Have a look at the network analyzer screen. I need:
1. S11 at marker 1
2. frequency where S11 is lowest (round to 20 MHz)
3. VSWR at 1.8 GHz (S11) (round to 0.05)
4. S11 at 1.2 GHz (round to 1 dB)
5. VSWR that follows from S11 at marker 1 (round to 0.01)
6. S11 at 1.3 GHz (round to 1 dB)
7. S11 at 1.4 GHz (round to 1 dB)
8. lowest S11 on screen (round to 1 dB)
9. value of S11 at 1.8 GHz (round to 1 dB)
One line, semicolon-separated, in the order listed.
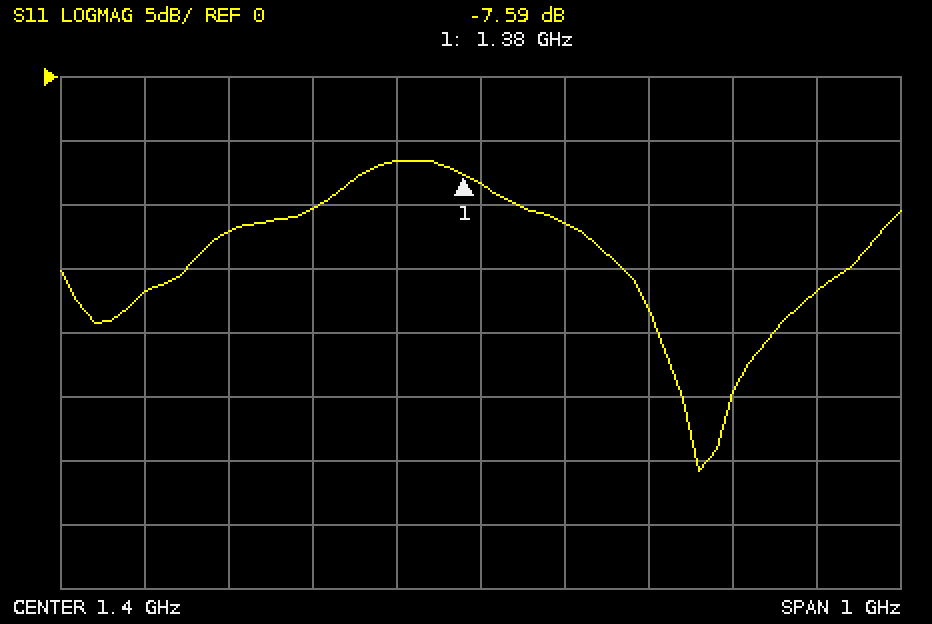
-7.59 dB; 1.66 GHz; 1.35; -10 dB; 2.43; -7 dB; -8 dB; -31 dB; -17 dB
